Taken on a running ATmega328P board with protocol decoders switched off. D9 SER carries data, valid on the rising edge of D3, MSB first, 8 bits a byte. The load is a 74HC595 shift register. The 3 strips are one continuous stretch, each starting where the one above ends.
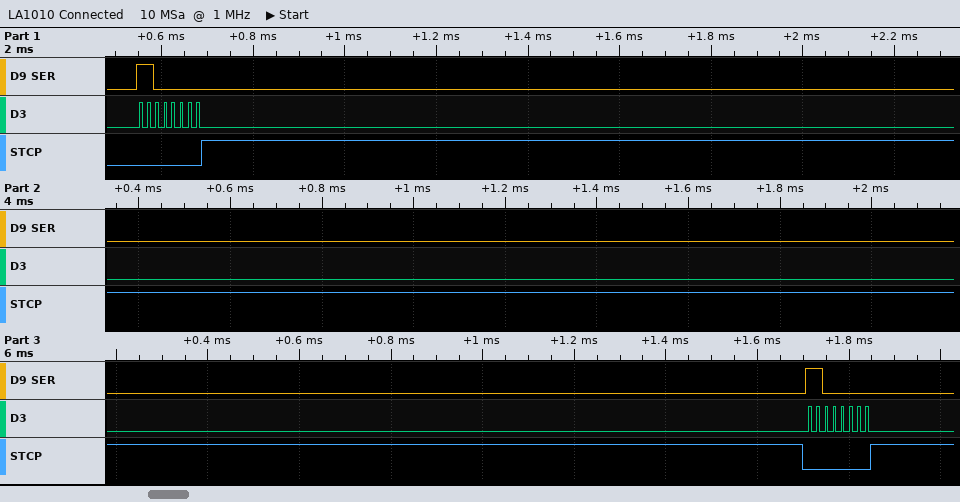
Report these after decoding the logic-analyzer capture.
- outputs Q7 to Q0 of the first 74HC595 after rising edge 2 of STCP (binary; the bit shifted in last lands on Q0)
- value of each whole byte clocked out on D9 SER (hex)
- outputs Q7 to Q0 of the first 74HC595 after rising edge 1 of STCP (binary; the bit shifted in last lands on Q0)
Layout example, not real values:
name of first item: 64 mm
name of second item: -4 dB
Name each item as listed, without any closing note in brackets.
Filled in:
outputs Q7 to Q0 of the first 74HC595 after rising edge 2 of STCP: 11000000
value of each whole byte clocked out on D9 SER: 0xC0 0xC0
outputs Q7 to Q0 of the first 74HC595 after rising edge 1 of STCP: 11000000
